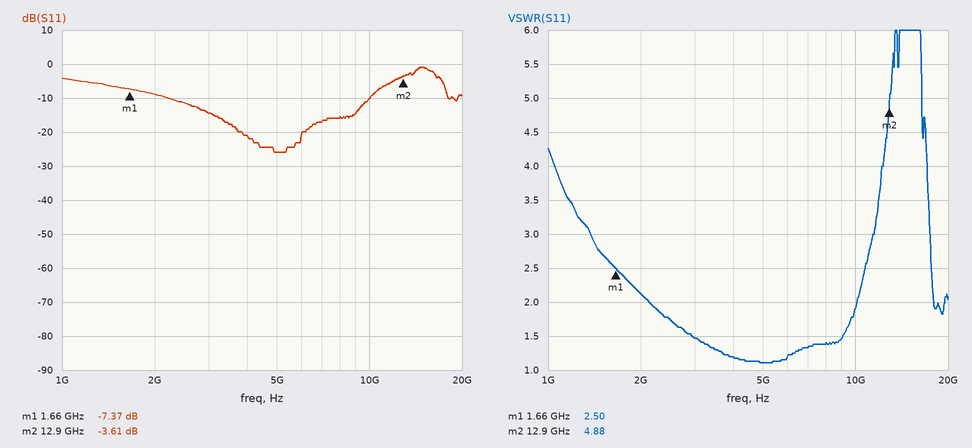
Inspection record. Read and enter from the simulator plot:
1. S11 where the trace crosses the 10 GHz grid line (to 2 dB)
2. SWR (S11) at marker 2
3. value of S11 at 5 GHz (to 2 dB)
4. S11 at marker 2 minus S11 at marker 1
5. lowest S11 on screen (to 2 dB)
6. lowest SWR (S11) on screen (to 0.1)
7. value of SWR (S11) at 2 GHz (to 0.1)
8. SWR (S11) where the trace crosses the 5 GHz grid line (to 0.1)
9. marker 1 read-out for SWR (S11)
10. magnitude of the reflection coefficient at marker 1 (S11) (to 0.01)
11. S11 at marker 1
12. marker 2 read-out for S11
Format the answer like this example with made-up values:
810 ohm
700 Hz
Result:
-10 dB
4.88
-26 dB
3.76 dB
-26 dB
1.1
2.1
1.1
2.50
0.43
-7.37 dB
-3.61 dB
